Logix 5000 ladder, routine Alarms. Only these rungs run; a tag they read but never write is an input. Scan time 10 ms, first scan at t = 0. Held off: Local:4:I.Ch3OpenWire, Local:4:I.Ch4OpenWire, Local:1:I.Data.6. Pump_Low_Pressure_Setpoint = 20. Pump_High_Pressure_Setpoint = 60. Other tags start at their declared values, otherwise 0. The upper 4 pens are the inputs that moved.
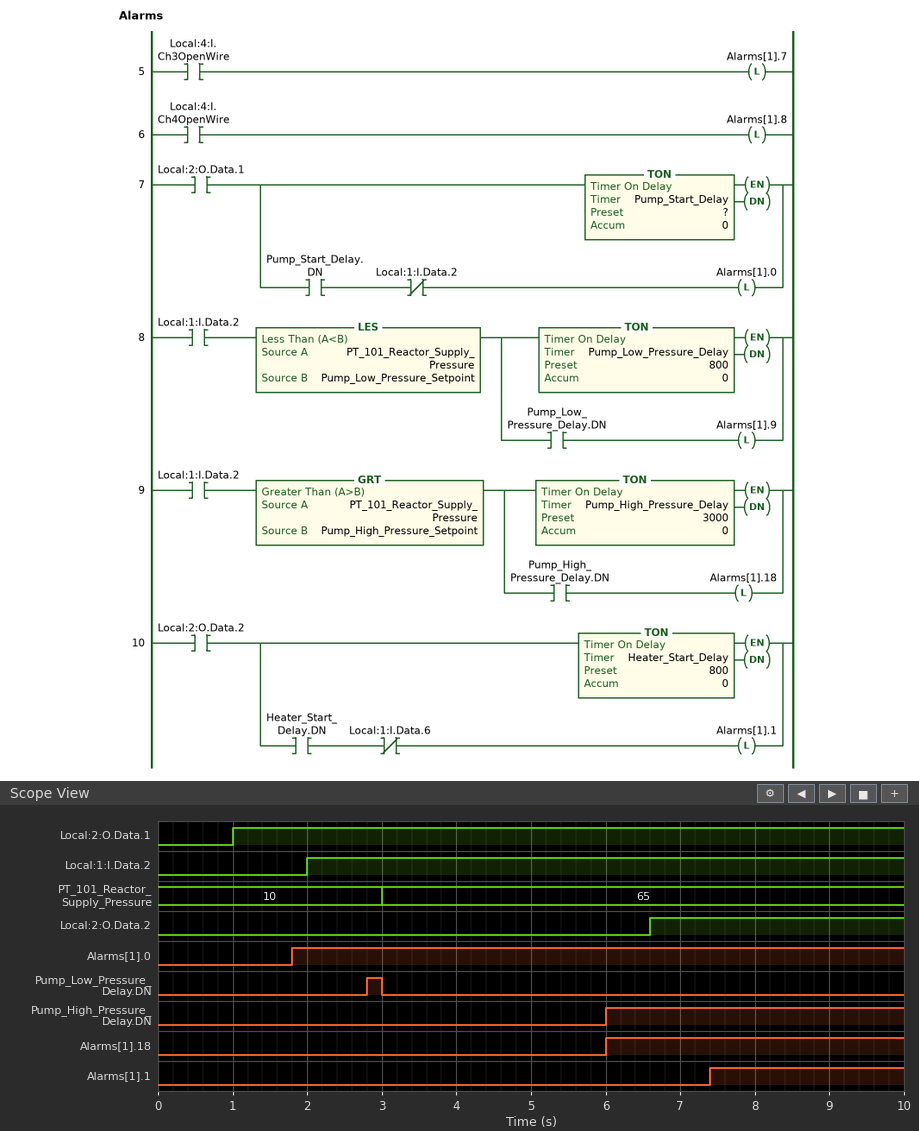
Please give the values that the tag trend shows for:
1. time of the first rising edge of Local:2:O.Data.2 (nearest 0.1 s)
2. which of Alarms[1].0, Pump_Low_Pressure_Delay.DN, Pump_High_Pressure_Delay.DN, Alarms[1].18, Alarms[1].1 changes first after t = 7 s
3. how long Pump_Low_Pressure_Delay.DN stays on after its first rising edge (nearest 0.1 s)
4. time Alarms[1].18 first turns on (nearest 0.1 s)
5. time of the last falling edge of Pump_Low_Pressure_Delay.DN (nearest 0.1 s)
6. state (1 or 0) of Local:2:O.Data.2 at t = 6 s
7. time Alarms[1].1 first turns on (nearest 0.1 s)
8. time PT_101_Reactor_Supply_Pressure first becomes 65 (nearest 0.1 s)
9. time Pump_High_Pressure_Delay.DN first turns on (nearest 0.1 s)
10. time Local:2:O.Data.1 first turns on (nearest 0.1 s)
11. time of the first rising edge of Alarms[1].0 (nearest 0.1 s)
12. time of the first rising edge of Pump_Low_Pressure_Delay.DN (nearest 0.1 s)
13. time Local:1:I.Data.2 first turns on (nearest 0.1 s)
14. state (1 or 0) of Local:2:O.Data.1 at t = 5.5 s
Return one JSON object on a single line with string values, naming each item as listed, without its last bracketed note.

{"time of the first rising edge of Local:2:O.Data.2": "6.6 s", "which of Alarms[1].0, Pump_Low_Pressure_Delay.DN, Pump_High_Pressure_Delay.DN, Alarms[1].18, Alarms[1].1 changes first after t = 7 s": "Alarms[1].1", "how long Pump_Low_Pressure_Delay.DN stays on after its first rising edge": "0.2 s", "time Alarms[1].18 first turns on": "6.0 s", "time of the last falling edge of Pump_Low_Pressure_Delay.DN": "3.0 s", "state (1 or 0) of Local:2:O.Data.2 at t = 6 s": "0", "time Alarms[1].1 first turns on": "7.4 s", "time PT_101_Reactor_Supply_Pressure first becomes 65": "3.0 s", "time Pump_High_Pressure_Delay.DN first turns on": "6.0 s", "time Local:2:O.Data.1 first turns on": "1.0 s", "time of the first rising edge of Alarms[1].0": "1.8 s", "time of the first rising edge of Pump_Low_Pressure_Delay.DN": "2.8 s", "time Local:1:I.Data.2 first turns on": "2.0 s", "state (1 or 0) of Local:2:O.Data.1 at t = 5.5 s": "1"}
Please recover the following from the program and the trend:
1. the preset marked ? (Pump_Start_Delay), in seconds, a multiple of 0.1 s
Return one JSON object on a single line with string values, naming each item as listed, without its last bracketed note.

{"the preset marked ? (Pump_Start_Delay), in seconds, a multiple of 0.1 s": "0.8 s"}
